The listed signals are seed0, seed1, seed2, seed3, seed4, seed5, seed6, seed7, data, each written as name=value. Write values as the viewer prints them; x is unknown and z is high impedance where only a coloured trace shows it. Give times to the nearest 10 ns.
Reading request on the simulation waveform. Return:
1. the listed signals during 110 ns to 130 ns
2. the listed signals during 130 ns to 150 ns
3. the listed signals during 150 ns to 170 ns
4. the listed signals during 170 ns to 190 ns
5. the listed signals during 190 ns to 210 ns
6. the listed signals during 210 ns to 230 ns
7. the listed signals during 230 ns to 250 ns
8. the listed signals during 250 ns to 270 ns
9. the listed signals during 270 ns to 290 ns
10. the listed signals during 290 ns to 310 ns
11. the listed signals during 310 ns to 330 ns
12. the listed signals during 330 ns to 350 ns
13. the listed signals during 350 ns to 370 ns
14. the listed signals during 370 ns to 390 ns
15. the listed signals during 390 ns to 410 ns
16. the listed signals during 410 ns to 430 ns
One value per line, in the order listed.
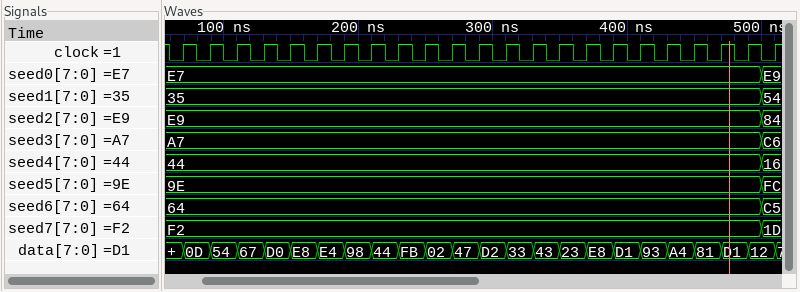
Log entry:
seed0=E7, seed1=35, seed2=E9, seed3=A7, seed4=44, seed5=9E, seed6=64, seed7=F2, data=67
seed0=E7, seed1=35, seed2=E9, seed3=A7, seed4=44, seed5=9E, seed6=64, seed7=F2, data=D0
seed0=E7, seed1=35, seed2=E9, seed3=A7, seed4=44, seed5=9E, seed6=64, seed7=F2, data=E8
seed0=E7, seed1=35, seed2=E9, seed3=A7, seed4=44, seed5=9E, seed6=64, seed7=F2, data=E4
seed0=E7, seed1=35, seed2=E9, seed3=A7, seed4=44, seed5=9E, seed6=64, seed7=F2, data=98
seed0=E7, seed1=35, seed2=E9, seed3=A7, seed4=44, seed5=9E, seed6=64, seed7=F2, data=44
seed0=E7, seed1=35, seed2=E9, seed3=A7, seed4=44, seed5=9E, seed6=64, seed7=F2, data=FB
seed0=E7, seed1=35, seed2=E9, seed3=A7, seed4=44, seed5=9E, seed6=64, seed7=F2, data=02
seed0=E7, seed1=35, seed2=E9, seed3=A7, seed4=44, seed5=9E, seed6=64, seed7=F2, data=47
seed0=E7, seed1=35, seed2=E9, seed3=A7, seed4=44, seed5=9E, seed6=64, seed7=F2, data=D2
seed0=E7, seed1=35, seed2=E9, seed3=A7, seed4=44, seed5=9E, seed6=64, seed7=F2, data=33
seed0=E7, seed1=35, seed2=E9, seed3=A7, seed4=44, seed5=9E, seed6=64, seed7=F2, data=43
seed0=E7, seed1=35, seed2=E9, seed3=A7, seed4=44, seed5=9E, seed6=64, seed7=F2, data=23
seed0=E7, seed1=35, seed2=E9, seed3=A7, seed4=44, seed5=9E, seed6=64, seed7=F2, data=E8
seed0=E7, seed1=35, seed2=E9, seed3=A7, seed4=44, seed5=9E, seed6=64, seed7=F2, data=D1
seed0=E7, seed1=35, seed2=E9, seed3=A7, seed4=44, seed5=9E, seed6=64, seed7=F2, data=93
